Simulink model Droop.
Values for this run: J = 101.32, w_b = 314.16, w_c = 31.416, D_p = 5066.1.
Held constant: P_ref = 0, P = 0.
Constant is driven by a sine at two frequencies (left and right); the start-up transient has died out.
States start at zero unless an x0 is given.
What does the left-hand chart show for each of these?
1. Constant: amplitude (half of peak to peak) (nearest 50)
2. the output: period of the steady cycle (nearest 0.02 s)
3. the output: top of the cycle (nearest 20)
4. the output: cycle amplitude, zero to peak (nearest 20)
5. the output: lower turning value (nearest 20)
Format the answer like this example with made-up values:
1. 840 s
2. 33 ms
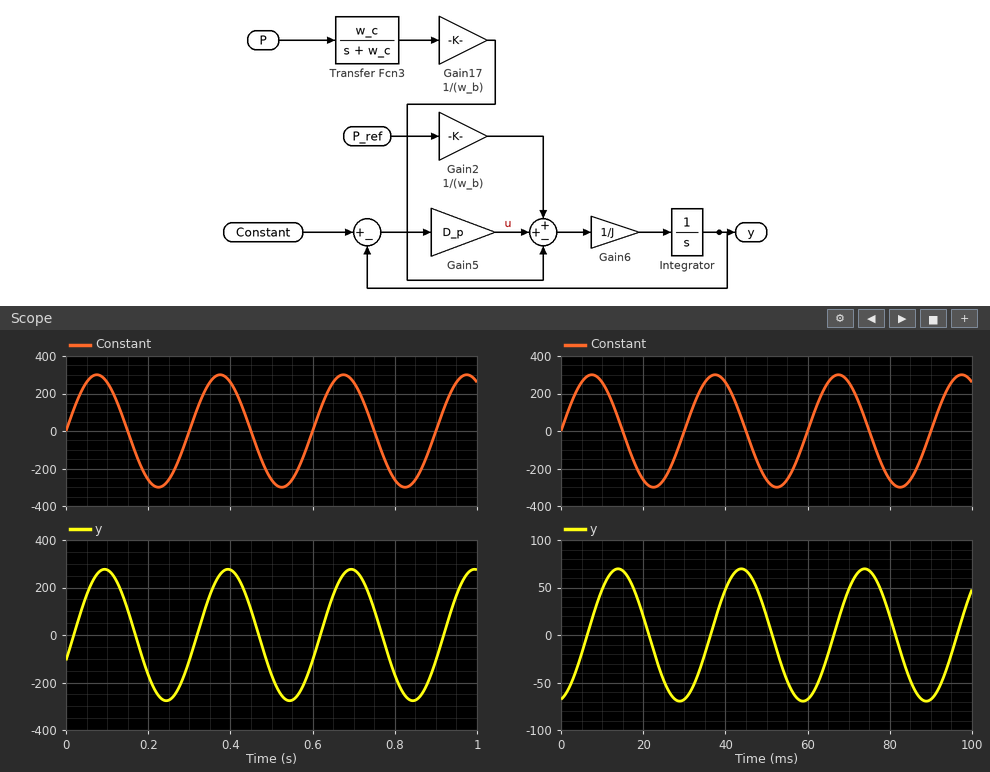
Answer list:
1. 300
2. 0.30 s
3. 280
4. 280
5. -280
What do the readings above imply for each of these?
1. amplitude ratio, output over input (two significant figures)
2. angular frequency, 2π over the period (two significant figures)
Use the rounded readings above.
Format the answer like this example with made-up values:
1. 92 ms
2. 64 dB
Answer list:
1. 0.93
2. 21 rad/s
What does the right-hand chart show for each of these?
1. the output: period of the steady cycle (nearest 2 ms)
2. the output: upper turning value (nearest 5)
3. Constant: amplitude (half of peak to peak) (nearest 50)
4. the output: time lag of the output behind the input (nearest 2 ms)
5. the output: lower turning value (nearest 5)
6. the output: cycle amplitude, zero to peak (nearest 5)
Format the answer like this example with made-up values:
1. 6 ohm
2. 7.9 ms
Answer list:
1. 30 ms
2. 70
3. 300
4. 6 ms
5. -70
6. 70
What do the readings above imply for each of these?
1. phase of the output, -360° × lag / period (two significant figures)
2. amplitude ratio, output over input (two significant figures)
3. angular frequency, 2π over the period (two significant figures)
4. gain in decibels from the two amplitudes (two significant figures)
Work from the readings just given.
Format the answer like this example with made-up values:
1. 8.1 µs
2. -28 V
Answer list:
1. -72°
2. 0.23
3. 0.21 rad/ms
4. -13 dB
